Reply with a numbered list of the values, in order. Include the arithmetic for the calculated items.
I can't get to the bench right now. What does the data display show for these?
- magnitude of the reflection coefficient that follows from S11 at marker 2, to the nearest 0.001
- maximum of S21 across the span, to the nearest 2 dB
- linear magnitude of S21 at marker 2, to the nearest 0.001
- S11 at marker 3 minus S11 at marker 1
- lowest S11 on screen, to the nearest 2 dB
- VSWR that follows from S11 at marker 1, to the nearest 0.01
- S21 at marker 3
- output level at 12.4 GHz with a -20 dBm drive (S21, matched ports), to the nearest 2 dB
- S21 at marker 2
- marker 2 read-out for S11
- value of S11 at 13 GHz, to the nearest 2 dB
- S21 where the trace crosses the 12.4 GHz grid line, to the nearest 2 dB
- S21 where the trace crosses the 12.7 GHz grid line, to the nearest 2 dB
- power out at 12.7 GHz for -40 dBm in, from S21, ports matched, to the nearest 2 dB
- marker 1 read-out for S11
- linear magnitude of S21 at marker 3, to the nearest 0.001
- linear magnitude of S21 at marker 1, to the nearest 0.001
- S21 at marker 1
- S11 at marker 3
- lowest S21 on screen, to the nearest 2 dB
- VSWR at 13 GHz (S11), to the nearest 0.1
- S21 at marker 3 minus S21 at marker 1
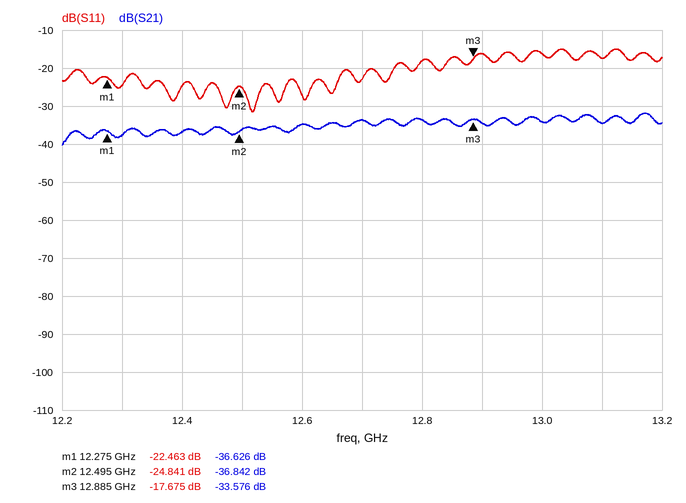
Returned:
1. 10^(-24.841/20) ≈ 0.057
2. -32 dB
3. 10^(-36.842/20) ≈ 0.014
4. -17.675 − (-22.463) = 4.788 dB
5. -32 dB
6. (1 + 0.0753)/(1 − 0.0753) ≈ 1.16
7. -33.576 dB
8. -20 dBm + (-36 dB) = -56 dBm
9. -36.842 dB
10. -24.841 dB
11. -16 dB
12. -36 dB
13. -34 dB
14. -40 dBm + (-34 dB) = -74 dBm
15. -22.463 dB
16. 10^(-33.576/20) ≈ 0.021
17. 10^(-36.626/20) ≈ 0.015
18. -36.626 dB
19. -17.675 dB
20. -40 dB
21. |Γ| = 10^(-16/20) = 0.1585; VSWR = (1 + 0.1585)/(1 − 0.1585) ≈ 1.4
22. -33.576 − (-36.626) = 3.050 dB
